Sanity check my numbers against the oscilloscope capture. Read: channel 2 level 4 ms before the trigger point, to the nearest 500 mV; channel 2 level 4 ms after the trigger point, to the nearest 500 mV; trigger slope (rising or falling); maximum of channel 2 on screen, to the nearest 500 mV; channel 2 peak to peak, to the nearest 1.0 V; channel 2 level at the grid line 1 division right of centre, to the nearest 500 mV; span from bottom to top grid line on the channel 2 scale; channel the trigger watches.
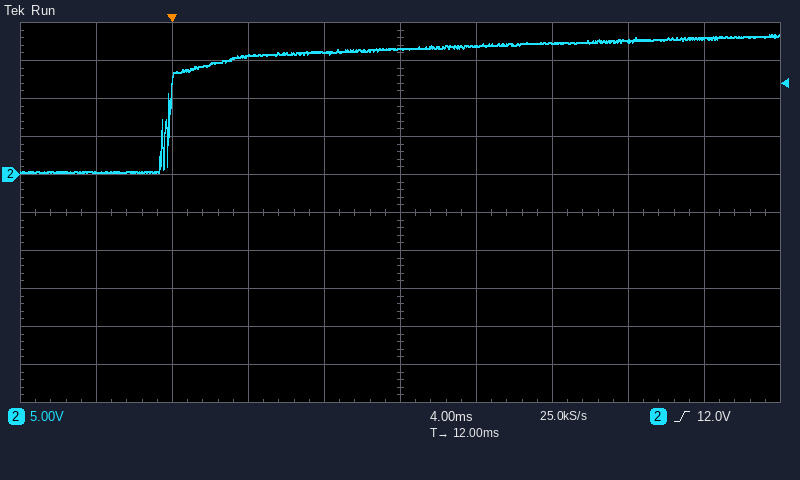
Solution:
500 mV
15.5 V
rising
18.5 V
18.0 V
17.0 V
50 V
channel 2
